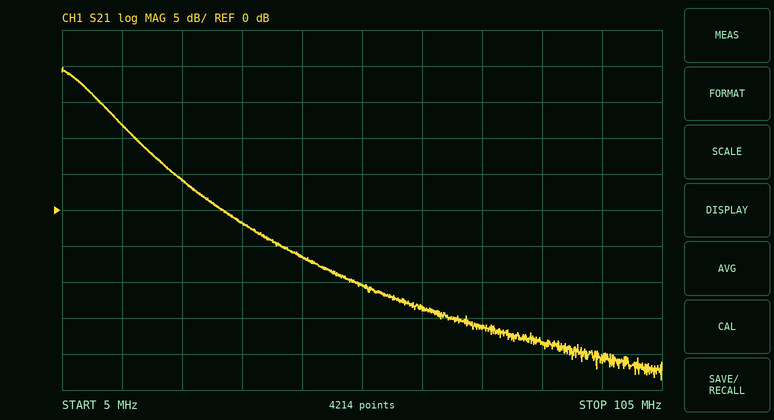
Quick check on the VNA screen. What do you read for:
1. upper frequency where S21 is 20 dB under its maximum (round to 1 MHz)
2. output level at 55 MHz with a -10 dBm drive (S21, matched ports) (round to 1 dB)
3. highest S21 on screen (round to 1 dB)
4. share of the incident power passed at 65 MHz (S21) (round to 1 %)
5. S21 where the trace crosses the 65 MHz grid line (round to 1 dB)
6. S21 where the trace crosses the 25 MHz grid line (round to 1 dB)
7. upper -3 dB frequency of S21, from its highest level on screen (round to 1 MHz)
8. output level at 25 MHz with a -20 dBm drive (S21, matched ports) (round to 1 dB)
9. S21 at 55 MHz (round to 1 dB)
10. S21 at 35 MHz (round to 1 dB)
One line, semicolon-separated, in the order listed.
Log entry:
32 MHz; -20 dBm; 20 dB; 4 %; -14 dB; 4 dB; 9 MHz; -16 dBm; -10 dB; -2 dB
